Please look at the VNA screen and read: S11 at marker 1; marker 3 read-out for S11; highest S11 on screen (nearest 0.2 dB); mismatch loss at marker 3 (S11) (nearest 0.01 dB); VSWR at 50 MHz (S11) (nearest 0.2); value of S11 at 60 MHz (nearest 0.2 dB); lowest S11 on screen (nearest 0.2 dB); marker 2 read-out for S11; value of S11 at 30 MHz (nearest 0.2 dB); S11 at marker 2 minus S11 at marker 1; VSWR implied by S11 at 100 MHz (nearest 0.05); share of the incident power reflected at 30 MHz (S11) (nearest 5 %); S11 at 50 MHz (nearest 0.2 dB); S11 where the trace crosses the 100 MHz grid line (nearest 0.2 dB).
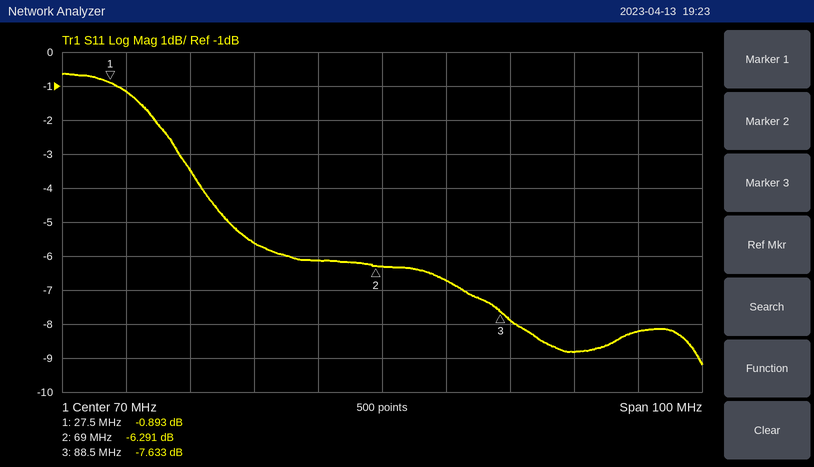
-0.893 dB
-7.633 dB
-0.6 dB
0.82 dB
3.2
-6.2 dB
-9.2 dB
-6.291 dB
-1.2 dB
-5.398 dB
2.15
75 %
-5.6 dB
-8.8 dB
